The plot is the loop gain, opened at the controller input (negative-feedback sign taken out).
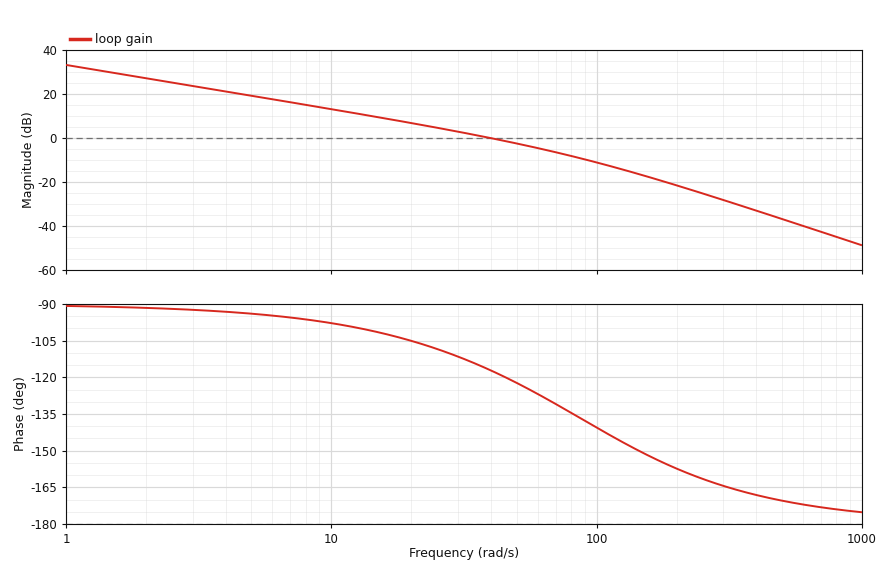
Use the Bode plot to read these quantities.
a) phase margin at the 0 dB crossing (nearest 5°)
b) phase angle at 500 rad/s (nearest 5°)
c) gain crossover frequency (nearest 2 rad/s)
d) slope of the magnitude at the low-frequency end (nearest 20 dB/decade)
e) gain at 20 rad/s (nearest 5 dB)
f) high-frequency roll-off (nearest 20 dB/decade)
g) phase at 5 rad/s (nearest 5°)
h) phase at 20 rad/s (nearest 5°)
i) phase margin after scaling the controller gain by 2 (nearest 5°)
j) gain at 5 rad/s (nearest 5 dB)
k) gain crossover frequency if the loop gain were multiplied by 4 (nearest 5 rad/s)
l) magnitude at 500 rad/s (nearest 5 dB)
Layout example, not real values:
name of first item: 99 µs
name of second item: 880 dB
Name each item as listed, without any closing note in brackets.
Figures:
phase margin at the 0 dB crossing: 65°
phase angle at 500 rad/s: -170°
gain crossover frequency: 40 rad/s
slope of the magnitude at the low-frequency end: -20 dB/decade
gain at 20 rad/s: 5 dB
high-frequency roll-off: -40 dB/decade
phase at 5 rad/s: -95°
phase at 20 rad/s: -105°
phase margin after scaling the controller gain by 2: 50°
gain at 5 rad/s: 20 dB
gain crossover frequency if the loop gain were multiplied by 4: 105 rad/s
magnitude at 500 rad/s: -35 dB
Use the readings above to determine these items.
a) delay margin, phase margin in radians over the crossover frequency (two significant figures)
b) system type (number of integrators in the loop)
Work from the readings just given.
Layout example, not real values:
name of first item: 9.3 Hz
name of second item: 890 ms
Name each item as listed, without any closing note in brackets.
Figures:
delay margin, phase margin in radians over the crossover frequency: 0.028 s
system type: 1
